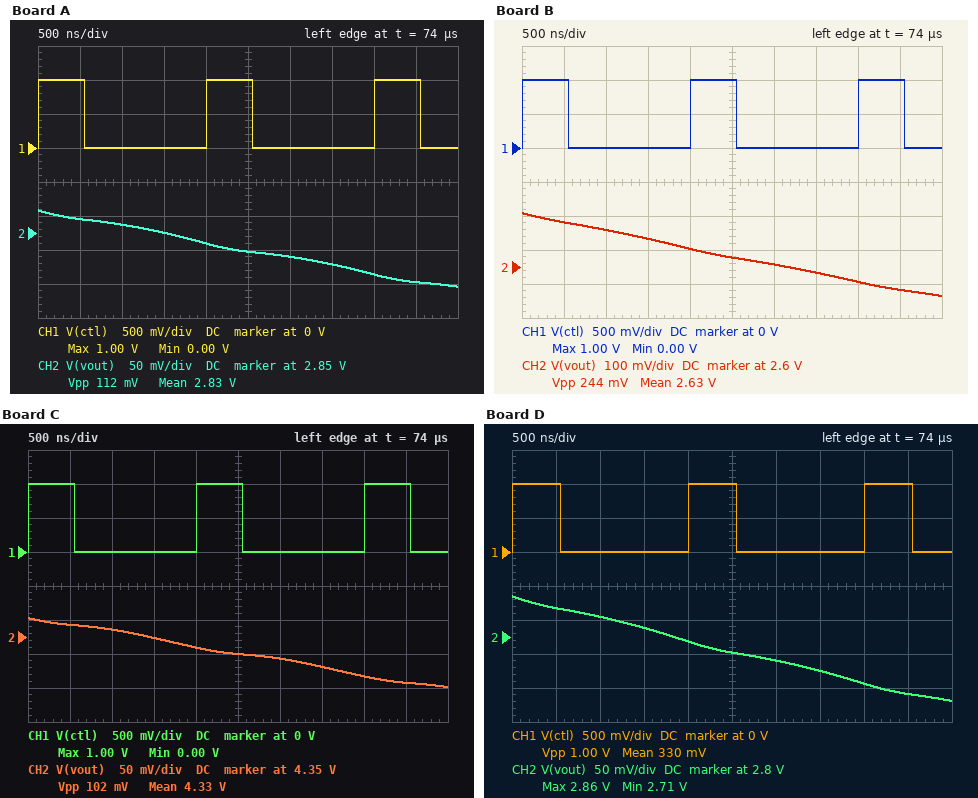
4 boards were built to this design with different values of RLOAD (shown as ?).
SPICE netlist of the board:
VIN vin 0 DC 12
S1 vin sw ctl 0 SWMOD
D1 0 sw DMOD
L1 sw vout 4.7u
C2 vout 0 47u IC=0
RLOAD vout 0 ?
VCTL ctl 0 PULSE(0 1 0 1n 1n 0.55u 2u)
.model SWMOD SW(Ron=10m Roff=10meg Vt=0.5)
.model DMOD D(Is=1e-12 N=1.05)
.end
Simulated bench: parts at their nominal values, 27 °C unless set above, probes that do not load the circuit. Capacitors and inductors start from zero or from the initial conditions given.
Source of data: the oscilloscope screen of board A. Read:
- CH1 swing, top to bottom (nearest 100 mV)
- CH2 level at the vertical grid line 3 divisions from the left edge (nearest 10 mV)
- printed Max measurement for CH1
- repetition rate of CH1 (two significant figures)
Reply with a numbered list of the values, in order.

1. 1.0 V
2. 2.85 V
3. 1.00 V
4. 500 kHz
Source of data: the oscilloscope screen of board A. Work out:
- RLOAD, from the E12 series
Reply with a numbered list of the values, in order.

1. 0.39 Ω
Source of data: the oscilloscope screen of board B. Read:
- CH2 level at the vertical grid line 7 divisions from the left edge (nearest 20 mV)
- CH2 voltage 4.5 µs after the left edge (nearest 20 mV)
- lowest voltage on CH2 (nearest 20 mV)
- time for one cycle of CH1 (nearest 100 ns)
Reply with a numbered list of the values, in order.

1. 2.58 V
2. 2.54 V
3. 2.52 V
4. 2.0 µs
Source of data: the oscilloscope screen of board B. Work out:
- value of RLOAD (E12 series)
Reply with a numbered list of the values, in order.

1. 0.68 Ω
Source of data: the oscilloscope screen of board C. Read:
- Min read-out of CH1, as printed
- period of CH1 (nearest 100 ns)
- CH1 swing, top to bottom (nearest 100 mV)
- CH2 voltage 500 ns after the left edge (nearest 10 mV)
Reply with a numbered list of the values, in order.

1. 0.00 V
2. 2.0 µs
3. 1.0 V
4. 4.37 V
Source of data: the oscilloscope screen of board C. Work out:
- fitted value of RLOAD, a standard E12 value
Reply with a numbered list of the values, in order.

1. 3.3 Ω
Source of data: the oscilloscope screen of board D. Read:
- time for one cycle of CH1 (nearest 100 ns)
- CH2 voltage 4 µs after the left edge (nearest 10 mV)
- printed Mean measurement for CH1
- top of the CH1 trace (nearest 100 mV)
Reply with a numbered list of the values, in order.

1. 2.0 µs
2. 2.73 V
3. 330 mV
4. 1.0 V
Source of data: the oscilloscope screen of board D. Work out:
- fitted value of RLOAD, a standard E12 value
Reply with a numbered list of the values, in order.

1. 0.47 Ω
